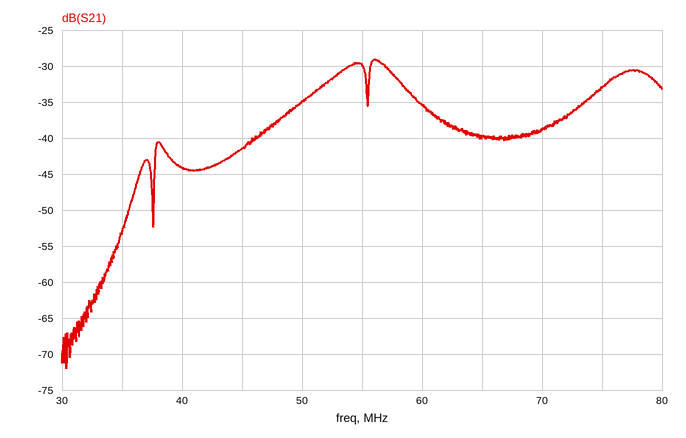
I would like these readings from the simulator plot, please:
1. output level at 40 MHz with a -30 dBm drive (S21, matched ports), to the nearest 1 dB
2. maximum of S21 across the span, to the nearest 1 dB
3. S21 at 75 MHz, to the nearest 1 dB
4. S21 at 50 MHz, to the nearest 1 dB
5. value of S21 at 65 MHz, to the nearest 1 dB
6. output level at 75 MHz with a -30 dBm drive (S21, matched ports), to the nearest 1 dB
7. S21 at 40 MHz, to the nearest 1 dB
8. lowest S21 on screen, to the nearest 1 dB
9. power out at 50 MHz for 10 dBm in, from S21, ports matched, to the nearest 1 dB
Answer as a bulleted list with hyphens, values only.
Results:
- -74 dBm
- -29 dB
- -33 dB
- -35 dB
- -40 dB
- -63 dBm
- -44 dB
- -72 dB
- -25 dBm
